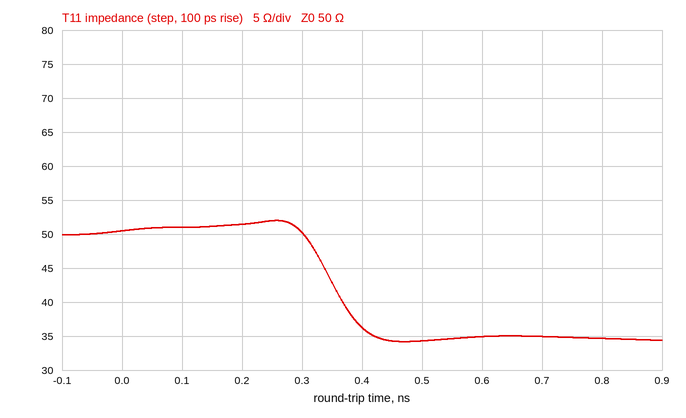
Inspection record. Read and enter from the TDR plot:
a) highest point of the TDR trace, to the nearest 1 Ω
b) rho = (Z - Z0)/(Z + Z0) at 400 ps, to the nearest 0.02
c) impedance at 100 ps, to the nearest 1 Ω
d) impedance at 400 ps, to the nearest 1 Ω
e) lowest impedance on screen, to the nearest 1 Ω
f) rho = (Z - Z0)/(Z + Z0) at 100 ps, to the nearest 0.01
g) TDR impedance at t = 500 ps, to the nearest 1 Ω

52 Ω
-0.16
51 Ω
36 Ω
34 Ω
+0.01
34 Ω
